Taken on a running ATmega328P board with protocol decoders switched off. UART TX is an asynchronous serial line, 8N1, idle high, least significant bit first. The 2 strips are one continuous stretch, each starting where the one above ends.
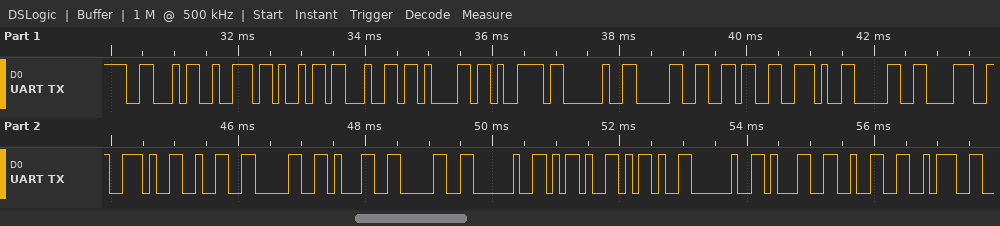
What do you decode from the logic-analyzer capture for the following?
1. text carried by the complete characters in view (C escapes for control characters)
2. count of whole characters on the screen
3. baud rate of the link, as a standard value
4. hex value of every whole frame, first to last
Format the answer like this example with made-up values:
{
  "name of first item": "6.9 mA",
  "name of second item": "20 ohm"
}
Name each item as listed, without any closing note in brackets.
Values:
{
  "text carried by the complete characters in view": "\"Friday 06.08.2010 -- 12:\"",
  "count of whole characters on the screen": "24",
  "baud rate of the link, as a standard value": "9600 baud",
  "hex value of every whole frame, first to last": "46 72 69 64 61 79 20 30 36 2E 30 38 2E 32 30 31 30 20 2D 2D 20 31 32 3A"
}
